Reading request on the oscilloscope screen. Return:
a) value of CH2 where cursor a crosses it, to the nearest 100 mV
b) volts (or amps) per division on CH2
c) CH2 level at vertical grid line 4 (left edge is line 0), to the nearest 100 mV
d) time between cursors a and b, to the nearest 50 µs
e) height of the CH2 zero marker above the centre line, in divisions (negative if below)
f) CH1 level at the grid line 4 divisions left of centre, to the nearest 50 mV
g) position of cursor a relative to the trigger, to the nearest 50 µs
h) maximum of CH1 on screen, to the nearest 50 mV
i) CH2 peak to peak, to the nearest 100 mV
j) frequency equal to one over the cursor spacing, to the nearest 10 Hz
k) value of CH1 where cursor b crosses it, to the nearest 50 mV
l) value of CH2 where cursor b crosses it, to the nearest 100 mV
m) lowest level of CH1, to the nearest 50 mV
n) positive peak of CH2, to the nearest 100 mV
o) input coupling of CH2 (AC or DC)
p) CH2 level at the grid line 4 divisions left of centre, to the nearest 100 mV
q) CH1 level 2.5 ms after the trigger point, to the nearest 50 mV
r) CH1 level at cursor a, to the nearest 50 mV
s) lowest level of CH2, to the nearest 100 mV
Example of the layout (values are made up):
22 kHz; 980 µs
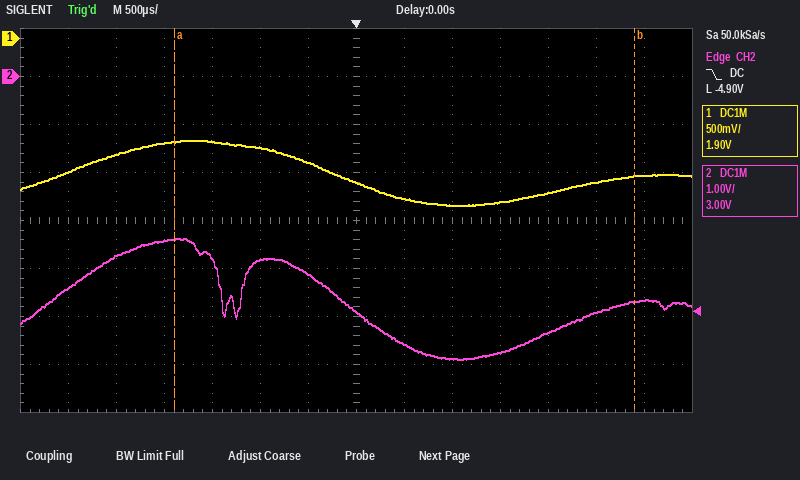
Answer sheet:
-3.4 V; 1 V; -3.8 V; 4.80 ms; +3.0 div; -1.10 V; -1.90 ms; -1.05 V; 2.5 V; 210 Hz; -1.45 V; -4.7 V; -1.75 V; -3.4 V; DC; -3.4 V; -1.50 V; -1.10 V; -5.9 V
